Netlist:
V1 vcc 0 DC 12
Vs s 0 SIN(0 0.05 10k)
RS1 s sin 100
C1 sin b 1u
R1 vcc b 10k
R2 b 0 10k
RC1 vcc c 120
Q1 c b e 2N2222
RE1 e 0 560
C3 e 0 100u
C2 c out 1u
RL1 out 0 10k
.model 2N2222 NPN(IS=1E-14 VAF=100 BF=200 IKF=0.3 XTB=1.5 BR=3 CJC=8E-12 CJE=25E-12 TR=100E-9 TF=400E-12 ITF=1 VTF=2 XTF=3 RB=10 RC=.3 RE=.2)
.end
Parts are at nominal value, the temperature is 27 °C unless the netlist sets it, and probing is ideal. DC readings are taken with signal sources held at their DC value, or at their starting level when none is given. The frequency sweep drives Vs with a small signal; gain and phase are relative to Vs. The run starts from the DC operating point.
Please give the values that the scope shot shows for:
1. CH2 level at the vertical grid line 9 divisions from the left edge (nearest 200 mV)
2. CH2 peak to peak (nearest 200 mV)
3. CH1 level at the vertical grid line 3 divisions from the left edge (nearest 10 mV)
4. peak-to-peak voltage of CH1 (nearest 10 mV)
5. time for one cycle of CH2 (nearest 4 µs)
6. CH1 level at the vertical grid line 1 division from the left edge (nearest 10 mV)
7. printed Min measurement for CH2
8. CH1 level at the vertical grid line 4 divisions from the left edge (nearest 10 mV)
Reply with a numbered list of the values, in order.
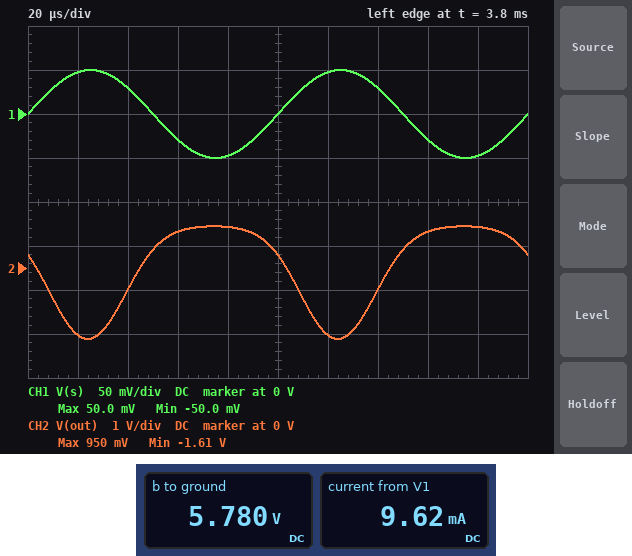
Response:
1. 1.0 V
2. 2.6 V
3. -30 mV
4. 100 mV
5. 100 µs
6. 50 mV
7. -1.61 V
8. -50 mV
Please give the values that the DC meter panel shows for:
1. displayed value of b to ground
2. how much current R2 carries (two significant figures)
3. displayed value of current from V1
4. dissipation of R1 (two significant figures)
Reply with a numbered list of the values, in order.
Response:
1. 5.780 V
2. 580 µA
3. 9.62 mA
4. 3.9 mW
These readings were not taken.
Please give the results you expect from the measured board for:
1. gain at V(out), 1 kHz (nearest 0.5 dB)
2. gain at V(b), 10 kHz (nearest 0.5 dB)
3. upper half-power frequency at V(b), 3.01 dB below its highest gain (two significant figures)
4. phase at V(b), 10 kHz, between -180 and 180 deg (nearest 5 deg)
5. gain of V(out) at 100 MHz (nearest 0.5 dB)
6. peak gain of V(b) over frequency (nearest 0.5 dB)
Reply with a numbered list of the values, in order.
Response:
1. 28.5 dB
2. -1.5 dB
3. 5.4 MHz
4. 0 deg
5. 4.5 dB
6. -1.5 dB
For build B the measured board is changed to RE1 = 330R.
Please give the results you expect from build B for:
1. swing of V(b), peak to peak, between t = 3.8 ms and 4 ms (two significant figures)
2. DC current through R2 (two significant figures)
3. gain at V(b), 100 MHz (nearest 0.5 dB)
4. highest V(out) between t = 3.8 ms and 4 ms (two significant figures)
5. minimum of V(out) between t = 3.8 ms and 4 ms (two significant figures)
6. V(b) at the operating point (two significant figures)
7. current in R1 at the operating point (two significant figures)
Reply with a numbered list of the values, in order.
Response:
1. 81 mV
2. 560 µA
3. -20.0 dB
4. 1.5 V
5. -2.2 V
6. 5.6 V
7. 640 µA
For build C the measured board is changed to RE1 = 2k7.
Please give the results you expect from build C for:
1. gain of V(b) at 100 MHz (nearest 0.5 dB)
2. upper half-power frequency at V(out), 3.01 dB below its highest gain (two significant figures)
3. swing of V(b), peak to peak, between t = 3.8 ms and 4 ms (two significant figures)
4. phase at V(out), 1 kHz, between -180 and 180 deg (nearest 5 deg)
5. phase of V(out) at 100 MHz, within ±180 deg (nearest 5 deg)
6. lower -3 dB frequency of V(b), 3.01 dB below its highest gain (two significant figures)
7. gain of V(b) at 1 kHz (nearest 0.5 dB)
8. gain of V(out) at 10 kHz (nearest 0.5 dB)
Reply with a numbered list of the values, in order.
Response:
1. -15.5 dB
2. 14 MHz
3. 95 mV
4. -170 deg
5. 85 deg
6. 78 Hz
7. -0.5 dB
8. 18.5 dB
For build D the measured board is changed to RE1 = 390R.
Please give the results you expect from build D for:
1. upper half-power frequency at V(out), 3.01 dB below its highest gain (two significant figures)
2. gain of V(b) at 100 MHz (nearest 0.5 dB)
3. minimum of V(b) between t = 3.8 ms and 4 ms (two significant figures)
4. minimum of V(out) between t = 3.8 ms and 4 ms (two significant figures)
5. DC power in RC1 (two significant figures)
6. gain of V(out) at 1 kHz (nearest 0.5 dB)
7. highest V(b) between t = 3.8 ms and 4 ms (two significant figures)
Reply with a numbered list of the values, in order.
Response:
1. 4.3 MHz
2. -20.0 dB
3. 5.6 V
4. -2.0 V
5. 19 mW
6. 29.5 dB
7. 5.7 V
